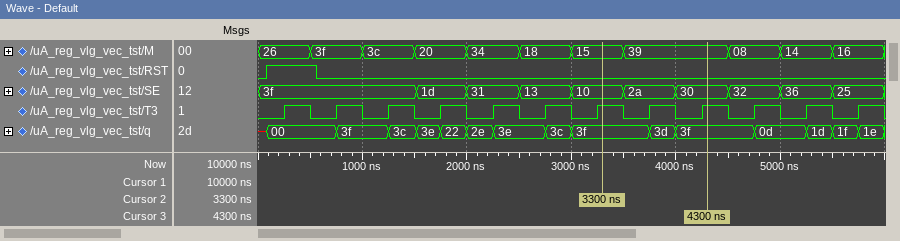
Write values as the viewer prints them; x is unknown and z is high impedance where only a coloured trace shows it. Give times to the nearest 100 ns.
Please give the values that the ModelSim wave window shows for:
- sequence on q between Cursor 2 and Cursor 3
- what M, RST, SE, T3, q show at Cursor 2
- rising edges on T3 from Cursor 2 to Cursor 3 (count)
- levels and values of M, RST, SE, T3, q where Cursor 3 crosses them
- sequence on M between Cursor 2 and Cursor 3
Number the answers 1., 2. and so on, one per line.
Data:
1. 3f, 3d, 3f
2. M=15, RST=0, SE=10, T3=1, q=3f
3. 2
4. M=39, RST=0, SE=30, T3=1, q=3f
5. 15, 39
